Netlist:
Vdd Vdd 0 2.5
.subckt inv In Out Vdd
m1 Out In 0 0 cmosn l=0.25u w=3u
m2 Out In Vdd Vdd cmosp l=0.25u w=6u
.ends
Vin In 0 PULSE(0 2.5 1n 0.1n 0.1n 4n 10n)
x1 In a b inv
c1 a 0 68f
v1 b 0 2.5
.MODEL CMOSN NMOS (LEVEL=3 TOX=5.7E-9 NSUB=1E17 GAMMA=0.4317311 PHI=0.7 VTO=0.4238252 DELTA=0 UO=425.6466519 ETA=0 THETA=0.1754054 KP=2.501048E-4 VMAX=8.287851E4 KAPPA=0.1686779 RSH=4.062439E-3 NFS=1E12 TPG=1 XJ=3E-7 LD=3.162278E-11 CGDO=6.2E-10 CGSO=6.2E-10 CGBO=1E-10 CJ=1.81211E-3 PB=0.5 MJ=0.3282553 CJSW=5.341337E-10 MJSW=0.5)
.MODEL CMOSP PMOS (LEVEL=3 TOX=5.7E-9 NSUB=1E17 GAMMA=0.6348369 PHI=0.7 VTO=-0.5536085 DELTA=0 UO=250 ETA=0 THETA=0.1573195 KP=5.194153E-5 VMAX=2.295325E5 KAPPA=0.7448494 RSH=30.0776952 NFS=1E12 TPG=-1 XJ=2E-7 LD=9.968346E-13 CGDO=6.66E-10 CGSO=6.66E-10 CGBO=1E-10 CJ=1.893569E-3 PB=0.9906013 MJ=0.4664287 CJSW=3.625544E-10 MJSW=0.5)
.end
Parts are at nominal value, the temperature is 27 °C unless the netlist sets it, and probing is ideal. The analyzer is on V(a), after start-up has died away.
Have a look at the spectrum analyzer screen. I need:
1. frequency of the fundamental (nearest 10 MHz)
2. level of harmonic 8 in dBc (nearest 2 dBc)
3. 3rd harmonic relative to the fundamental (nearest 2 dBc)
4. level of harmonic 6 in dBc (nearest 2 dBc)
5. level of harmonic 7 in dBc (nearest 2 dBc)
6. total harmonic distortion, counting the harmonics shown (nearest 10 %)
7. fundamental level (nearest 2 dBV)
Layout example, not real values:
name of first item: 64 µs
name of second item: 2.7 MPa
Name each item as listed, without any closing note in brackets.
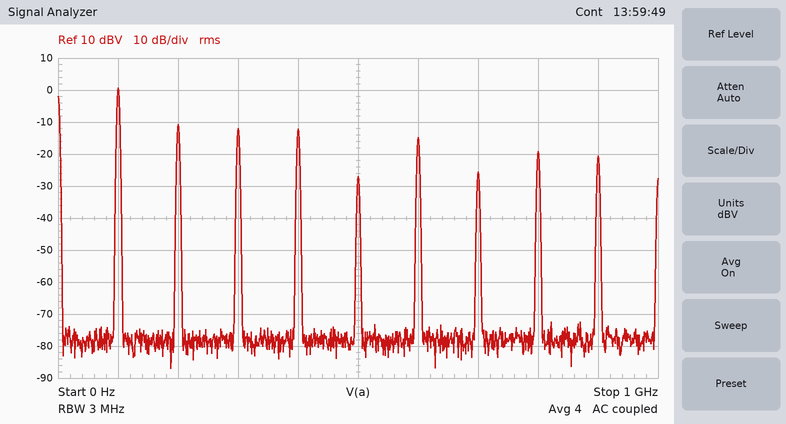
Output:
frequency of the fundamental: 100 MHz
level of harmonic 8 in dBc: -20 dBc
3rd harmonic relative to the fundamental: -12 dBc
level of harmonic 6 in dBc: -16 dBc
level of harmonic 7 in dBc: -26 dBc
total harmonic distortion, counting the harmonics shown: 50 %
fundamental level: 0 dBV
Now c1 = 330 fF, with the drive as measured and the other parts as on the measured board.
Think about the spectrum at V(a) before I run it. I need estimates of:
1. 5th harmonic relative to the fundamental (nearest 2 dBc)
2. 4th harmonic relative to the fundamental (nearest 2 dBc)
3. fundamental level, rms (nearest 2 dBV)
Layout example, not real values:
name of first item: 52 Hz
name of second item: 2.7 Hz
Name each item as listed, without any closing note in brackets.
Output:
5th harmonic relative to the fundamental: -26 dBc
4th harmonic relative to the fundamental: -14 dBc
fundamental level, rms: 0 dBV
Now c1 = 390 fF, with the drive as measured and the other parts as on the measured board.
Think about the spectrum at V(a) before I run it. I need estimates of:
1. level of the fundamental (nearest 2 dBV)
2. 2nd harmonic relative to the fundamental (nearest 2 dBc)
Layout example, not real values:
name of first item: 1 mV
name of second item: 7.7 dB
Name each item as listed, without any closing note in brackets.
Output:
level of the fundamental: 0 dBV
2nd harmonic relative to the fundamental: -12 dBc
